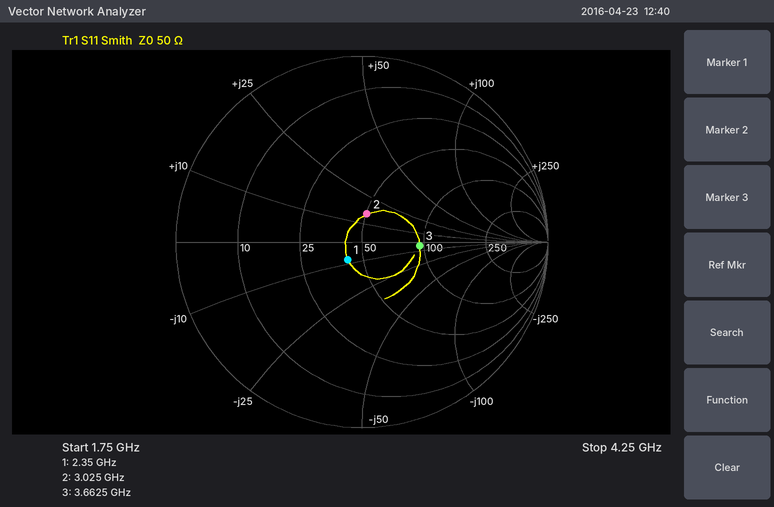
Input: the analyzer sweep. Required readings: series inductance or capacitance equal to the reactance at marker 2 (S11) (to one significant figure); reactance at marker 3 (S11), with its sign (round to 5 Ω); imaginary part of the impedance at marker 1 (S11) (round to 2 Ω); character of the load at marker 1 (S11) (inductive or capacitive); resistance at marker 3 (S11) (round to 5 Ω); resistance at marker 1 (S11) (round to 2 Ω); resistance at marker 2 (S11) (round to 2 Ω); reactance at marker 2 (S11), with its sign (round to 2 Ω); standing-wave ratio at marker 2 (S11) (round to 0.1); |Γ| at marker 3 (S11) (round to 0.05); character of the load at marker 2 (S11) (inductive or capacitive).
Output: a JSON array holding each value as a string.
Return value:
["800 pH", "-5 Ω", "-8 Ω", "capacitive", "95 Ω", "42 Ω", "50 Ω", "+16 Ω", "1.4", "0.30", "inductive"]
